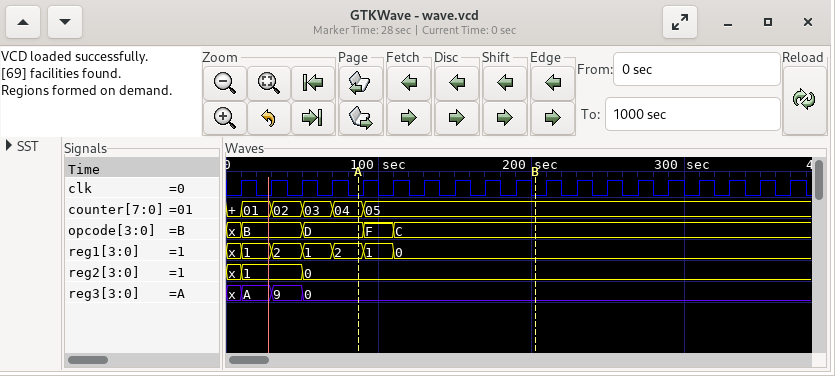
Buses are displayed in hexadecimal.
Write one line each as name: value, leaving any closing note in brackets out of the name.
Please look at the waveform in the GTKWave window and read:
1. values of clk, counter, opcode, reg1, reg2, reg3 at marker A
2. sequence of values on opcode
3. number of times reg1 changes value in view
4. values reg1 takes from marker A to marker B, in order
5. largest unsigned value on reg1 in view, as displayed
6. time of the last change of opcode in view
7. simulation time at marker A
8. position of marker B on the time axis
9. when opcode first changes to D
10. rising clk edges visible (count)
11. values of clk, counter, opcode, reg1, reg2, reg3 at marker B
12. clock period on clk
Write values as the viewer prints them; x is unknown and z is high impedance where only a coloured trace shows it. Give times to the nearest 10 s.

values of clk, counter, opcode, reg1, reg2, reg3 at marker A: clk=0, counter=04, opcode=D, reg1=2, reg2=0, reg3=0
sequence of values on opcode: x, B, D, F, C
number of times reg1 changes value in view: 6
values reg1 takes from marker A to marker B, in order: 2, 1, 0
largest unsigned value on reg1 in view, as displayed: 2
time of the last change of opcode in view: 110 s
simulation time at marker A: 90 s
position of marker B on the time axis: 200 s
when opcode first changes to D: 50 s
rising clk edges visible: 19
values of clk, counter, opcode, reg1, reg2, reg3 at marker B: clk=0, counter=05, opcode=C, reg1=0, reg2=0, reg3=0
clock period on clk: 20 s
